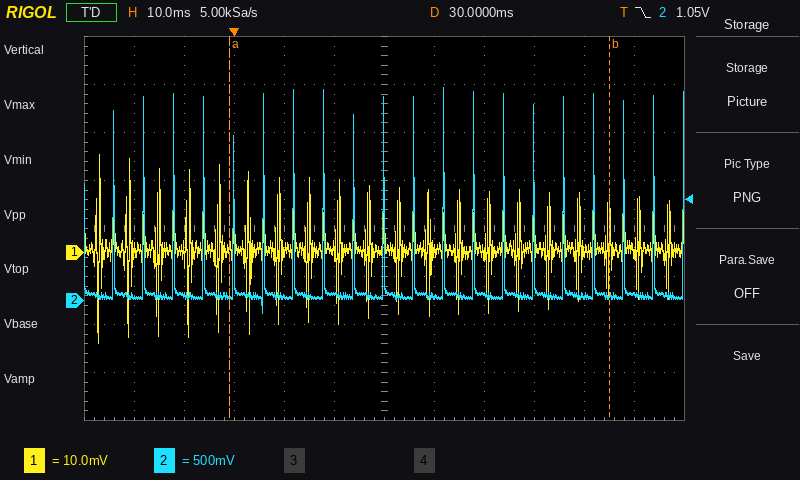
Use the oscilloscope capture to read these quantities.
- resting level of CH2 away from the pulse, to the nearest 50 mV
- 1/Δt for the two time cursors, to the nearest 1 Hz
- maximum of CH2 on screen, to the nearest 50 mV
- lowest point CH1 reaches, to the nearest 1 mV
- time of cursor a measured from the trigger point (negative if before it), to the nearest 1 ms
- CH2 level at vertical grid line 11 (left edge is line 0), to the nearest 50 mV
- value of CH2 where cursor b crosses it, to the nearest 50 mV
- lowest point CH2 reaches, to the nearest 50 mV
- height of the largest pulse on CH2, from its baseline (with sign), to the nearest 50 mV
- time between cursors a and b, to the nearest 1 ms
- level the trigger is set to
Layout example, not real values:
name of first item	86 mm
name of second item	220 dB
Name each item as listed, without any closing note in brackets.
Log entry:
resting level of CH2 away from the pulse, to the nearest 50 mV	50 mV
1/Δt for the two time cursors, to the nearest 1 Hz	13 Hz
maximum of CH2 on screen, to the nearest 50 mV	2.20 V
lowest point CH1 reaches, to the nearest 1 mV	-19 mV
time of cursor a measured from the trigger point (negative if before it), to the nearest 1 ms	-1 ms
CH2 level at vertical grid line 11 (left edge is line 0), to the nearest 50 mV	50 mV
value of CH2 where cursor b crosses it, to the nearest 50 mV	50 mV
lowest point CH2 reaches, to the nearest 50 mV	-100 mV
height of the largest pulse on CH2, from its baseline (with sign), to the nearest 50 mV	+2.15 V
time between cursors a and b, to the nearest 1 ms	76 ms
level the trigger is set to	1.05 V
